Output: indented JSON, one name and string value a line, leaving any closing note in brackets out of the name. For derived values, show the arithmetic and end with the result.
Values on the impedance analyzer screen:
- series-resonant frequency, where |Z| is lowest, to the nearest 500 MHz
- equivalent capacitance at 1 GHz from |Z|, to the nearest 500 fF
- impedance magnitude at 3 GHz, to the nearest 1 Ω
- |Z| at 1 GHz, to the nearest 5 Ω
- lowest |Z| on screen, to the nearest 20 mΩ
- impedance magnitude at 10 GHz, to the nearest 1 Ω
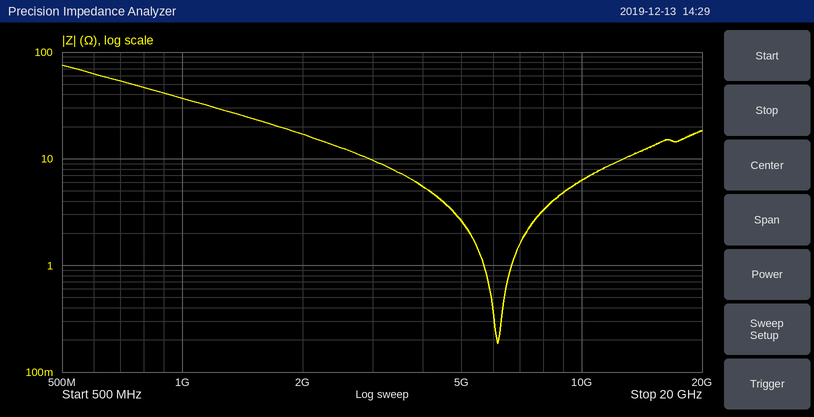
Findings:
{
  "series-resonant frequency, where |Z| is lowest, to the nearest 500 MHz": "6.0 GHz",
  "equivalent capacitance at 1 GHz from |Z|, to the nearest 500 fF": "C = 1/(2π × 1 GHz × 35 Ω) ≈ 4.5 pF",
  "impedance magnitude at 3 GHz, to the nearest 1 Ω": "10 Ω",
  "|Z| at 1 GHz, to the nearest 5 Ω": "35 Ω",
  "lowest |Z| on screen, to the nearest 20 mΩ": "180 mΩ",
  "impedance magnitude at 10 GHz, to the nearest 1 Ω": "6 Ω"
}
